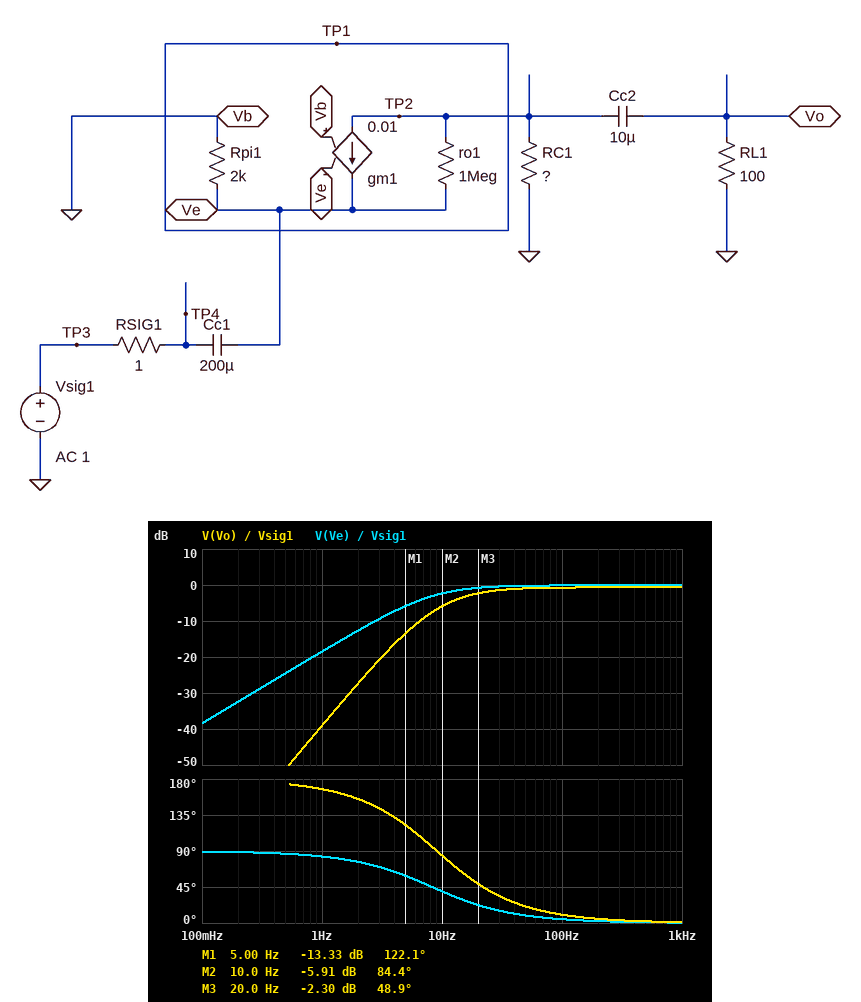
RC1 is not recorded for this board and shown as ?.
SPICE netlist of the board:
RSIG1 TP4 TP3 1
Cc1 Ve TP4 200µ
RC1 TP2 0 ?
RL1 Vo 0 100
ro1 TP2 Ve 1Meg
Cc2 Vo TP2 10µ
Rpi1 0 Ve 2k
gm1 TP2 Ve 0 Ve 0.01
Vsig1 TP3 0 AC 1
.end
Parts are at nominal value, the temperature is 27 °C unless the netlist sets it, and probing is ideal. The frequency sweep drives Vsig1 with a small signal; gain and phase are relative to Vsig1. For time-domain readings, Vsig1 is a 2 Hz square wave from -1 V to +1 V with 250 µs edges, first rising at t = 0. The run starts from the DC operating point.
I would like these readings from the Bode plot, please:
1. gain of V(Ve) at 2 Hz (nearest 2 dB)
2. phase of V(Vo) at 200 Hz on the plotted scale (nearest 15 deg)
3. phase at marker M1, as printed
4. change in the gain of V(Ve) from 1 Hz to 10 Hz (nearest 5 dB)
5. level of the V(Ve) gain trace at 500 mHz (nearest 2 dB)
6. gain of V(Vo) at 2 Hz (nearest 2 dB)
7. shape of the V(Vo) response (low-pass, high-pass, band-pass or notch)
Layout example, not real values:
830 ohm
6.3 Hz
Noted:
-12 dB
0 deg
122.1 deg
15 dB
-24 dB
-28 dB
high-pass
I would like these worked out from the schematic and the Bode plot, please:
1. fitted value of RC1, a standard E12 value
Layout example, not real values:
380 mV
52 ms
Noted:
1.5 kΩ
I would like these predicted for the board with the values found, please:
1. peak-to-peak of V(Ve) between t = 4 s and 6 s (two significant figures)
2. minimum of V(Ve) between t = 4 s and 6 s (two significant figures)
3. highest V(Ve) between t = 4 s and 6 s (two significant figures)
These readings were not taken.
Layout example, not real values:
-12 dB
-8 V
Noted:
3.9 V
-2.0 V
2.0 V
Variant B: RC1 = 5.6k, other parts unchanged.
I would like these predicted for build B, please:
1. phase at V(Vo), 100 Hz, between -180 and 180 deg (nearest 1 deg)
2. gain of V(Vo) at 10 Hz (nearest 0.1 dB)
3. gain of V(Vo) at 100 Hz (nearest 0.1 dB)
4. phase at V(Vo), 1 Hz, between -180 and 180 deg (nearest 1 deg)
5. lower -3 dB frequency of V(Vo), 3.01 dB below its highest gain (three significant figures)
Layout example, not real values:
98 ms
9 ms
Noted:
6 deg
-2.8 dB
-0.3 dB
153 deg
9.11 Hz
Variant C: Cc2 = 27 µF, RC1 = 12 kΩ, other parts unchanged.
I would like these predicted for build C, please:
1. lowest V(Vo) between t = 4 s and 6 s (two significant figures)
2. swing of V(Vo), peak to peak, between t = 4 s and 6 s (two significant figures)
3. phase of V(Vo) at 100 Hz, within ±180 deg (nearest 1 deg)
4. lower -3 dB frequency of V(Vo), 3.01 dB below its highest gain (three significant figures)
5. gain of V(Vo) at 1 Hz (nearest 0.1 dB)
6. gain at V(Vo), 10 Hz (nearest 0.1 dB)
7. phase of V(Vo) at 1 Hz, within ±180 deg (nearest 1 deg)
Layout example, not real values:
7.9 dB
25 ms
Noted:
-2.0 V
4.0 V
5 deg
8.30 Hz
-19.5 dB
-2.4 dB
109 deg
